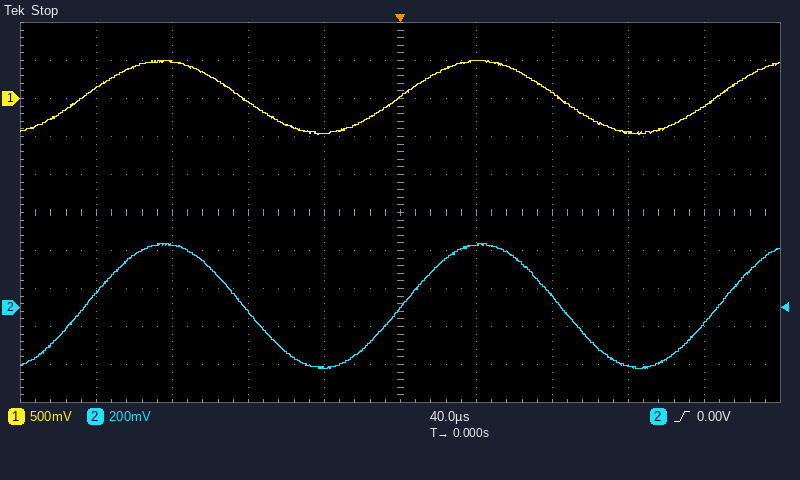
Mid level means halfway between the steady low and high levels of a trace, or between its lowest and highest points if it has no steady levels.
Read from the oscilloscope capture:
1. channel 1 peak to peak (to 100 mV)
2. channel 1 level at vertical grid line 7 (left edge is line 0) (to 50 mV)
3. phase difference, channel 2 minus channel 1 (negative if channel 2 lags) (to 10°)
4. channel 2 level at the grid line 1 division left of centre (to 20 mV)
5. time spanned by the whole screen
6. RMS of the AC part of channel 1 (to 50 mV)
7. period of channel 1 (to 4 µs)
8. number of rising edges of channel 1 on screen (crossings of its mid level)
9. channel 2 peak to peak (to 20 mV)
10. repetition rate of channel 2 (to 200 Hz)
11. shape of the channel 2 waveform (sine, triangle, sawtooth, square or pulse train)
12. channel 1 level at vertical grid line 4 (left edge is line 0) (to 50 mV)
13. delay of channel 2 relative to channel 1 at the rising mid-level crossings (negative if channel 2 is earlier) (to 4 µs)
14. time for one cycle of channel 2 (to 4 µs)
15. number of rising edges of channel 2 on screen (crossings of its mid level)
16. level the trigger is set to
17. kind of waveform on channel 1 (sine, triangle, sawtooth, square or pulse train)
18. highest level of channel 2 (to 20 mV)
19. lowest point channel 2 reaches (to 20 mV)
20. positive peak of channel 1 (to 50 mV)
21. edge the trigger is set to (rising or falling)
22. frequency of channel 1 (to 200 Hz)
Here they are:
1.00 V
100 mV
0°
-320 mV
400 µs
350 mV
168 µs
3
660 mV
6.0 kHz
sine
-450 mV
0 µs
168 µs
3
0.00 V
sine
340 mV
-320 mV
500 mV
rising
6.0 kHz
